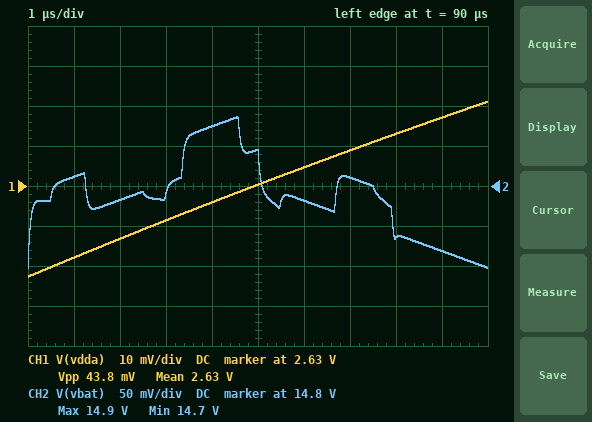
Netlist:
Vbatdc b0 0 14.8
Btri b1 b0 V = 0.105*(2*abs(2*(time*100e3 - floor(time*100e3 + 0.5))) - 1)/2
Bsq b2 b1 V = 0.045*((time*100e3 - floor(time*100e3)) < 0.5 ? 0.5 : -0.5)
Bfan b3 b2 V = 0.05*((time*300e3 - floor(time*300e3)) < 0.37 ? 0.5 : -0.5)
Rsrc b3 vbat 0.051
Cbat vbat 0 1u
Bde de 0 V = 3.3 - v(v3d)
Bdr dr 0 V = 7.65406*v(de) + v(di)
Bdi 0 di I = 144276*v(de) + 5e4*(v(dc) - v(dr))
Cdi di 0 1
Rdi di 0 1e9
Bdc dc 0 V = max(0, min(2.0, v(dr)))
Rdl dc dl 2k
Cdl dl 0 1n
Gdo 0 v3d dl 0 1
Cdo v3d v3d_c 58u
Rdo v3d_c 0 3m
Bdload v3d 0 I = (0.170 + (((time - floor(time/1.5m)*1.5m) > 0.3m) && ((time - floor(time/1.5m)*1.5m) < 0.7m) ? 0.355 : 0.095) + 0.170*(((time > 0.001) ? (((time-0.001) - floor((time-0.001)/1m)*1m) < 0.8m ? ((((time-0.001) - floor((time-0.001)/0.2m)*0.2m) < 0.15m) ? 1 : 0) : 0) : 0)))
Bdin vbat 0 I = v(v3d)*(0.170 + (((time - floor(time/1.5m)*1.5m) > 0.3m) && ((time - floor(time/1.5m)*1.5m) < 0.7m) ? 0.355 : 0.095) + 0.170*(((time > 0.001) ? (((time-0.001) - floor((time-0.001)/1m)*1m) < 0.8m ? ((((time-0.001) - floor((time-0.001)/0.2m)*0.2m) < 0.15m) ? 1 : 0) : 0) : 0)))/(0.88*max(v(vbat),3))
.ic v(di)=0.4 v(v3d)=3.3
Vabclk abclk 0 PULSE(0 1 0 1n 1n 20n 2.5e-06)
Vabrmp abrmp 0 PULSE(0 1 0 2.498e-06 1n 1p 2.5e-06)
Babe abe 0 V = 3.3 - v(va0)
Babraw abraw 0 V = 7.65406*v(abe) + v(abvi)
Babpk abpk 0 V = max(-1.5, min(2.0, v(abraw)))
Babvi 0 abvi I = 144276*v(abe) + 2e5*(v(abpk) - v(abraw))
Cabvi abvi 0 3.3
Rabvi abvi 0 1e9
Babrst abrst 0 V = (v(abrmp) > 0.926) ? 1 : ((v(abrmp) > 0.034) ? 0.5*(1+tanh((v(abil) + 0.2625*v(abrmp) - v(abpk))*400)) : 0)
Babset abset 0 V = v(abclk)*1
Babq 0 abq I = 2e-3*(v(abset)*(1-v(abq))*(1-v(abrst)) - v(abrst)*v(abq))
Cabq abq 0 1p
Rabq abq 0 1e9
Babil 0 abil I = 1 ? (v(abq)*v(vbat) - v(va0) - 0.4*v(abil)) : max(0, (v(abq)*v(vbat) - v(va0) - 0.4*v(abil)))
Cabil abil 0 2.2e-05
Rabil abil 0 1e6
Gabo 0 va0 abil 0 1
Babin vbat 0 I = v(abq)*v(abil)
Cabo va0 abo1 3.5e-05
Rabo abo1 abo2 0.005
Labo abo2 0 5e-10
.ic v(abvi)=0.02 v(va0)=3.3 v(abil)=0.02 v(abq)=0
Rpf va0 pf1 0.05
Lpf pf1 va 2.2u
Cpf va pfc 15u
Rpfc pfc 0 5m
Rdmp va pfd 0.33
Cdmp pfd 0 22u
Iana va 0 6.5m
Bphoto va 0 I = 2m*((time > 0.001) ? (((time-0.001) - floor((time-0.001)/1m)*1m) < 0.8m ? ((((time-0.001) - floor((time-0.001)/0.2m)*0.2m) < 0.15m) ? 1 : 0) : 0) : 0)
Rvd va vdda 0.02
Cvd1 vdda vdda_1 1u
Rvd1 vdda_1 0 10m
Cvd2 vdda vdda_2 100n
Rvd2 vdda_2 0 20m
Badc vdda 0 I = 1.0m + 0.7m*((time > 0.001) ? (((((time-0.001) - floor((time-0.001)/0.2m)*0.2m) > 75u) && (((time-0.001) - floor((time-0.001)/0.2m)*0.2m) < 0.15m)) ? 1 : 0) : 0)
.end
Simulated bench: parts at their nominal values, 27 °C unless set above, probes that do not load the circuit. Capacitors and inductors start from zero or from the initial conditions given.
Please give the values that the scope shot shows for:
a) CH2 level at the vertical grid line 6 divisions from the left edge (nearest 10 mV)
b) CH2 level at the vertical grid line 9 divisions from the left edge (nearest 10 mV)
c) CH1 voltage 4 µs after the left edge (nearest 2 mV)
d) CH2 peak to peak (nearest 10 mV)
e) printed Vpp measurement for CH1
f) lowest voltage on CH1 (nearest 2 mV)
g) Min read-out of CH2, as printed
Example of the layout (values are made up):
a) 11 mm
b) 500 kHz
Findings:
a) 14.78 V
b) 14.72 V
c) 2.626 V
d) 190 mV
e) 43.8 mV
f) 2.608 V
g) 14.7 V
